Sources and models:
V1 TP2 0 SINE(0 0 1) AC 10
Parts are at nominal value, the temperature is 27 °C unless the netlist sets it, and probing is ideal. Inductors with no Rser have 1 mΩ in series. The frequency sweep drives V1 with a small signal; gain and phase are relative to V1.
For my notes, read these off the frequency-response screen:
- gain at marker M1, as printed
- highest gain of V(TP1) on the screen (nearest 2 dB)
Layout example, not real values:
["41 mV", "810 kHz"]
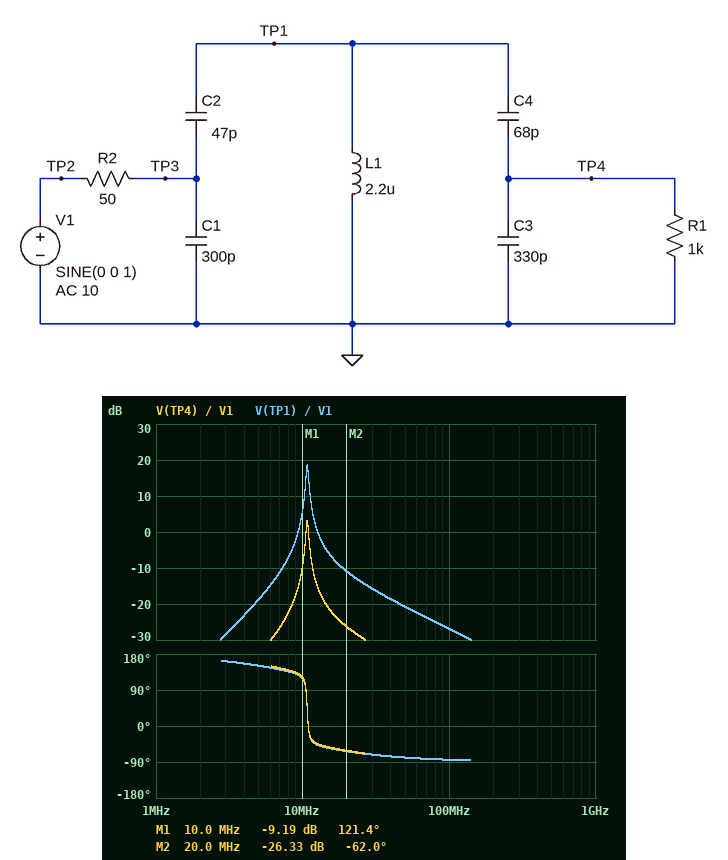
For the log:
["-9.19 dB", "18 dB"]
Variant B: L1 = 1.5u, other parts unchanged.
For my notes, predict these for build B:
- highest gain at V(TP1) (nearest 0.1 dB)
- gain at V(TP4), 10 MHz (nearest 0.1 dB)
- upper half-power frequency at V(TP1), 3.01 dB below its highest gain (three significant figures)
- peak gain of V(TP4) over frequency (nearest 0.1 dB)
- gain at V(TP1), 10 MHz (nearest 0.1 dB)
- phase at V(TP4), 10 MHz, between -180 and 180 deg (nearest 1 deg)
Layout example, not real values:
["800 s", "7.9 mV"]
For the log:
["18.1 dB", "-22.1 dB", "13.3 MHz", "2.8 dB", "-6.7 dB", "132 deg"]
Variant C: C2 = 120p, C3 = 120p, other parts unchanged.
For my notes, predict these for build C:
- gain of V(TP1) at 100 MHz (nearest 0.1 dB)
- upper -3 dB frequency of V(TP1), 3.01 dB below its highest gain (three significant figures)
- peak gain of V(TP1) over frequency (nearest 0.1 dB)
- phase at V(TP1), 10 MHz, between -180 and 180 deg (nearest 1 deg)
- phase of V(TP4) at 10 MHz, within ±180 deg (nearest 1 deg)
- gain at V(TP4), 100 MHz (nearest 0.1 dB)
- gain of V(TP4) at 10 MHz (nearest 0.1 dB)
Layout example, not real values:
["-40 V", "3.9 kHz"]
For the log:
["-23.0 dB", "9.62 MHz", "12.1 dB", "-18 deg", "-13 deg", "-31.8 dB", "-1.9 dB"]
